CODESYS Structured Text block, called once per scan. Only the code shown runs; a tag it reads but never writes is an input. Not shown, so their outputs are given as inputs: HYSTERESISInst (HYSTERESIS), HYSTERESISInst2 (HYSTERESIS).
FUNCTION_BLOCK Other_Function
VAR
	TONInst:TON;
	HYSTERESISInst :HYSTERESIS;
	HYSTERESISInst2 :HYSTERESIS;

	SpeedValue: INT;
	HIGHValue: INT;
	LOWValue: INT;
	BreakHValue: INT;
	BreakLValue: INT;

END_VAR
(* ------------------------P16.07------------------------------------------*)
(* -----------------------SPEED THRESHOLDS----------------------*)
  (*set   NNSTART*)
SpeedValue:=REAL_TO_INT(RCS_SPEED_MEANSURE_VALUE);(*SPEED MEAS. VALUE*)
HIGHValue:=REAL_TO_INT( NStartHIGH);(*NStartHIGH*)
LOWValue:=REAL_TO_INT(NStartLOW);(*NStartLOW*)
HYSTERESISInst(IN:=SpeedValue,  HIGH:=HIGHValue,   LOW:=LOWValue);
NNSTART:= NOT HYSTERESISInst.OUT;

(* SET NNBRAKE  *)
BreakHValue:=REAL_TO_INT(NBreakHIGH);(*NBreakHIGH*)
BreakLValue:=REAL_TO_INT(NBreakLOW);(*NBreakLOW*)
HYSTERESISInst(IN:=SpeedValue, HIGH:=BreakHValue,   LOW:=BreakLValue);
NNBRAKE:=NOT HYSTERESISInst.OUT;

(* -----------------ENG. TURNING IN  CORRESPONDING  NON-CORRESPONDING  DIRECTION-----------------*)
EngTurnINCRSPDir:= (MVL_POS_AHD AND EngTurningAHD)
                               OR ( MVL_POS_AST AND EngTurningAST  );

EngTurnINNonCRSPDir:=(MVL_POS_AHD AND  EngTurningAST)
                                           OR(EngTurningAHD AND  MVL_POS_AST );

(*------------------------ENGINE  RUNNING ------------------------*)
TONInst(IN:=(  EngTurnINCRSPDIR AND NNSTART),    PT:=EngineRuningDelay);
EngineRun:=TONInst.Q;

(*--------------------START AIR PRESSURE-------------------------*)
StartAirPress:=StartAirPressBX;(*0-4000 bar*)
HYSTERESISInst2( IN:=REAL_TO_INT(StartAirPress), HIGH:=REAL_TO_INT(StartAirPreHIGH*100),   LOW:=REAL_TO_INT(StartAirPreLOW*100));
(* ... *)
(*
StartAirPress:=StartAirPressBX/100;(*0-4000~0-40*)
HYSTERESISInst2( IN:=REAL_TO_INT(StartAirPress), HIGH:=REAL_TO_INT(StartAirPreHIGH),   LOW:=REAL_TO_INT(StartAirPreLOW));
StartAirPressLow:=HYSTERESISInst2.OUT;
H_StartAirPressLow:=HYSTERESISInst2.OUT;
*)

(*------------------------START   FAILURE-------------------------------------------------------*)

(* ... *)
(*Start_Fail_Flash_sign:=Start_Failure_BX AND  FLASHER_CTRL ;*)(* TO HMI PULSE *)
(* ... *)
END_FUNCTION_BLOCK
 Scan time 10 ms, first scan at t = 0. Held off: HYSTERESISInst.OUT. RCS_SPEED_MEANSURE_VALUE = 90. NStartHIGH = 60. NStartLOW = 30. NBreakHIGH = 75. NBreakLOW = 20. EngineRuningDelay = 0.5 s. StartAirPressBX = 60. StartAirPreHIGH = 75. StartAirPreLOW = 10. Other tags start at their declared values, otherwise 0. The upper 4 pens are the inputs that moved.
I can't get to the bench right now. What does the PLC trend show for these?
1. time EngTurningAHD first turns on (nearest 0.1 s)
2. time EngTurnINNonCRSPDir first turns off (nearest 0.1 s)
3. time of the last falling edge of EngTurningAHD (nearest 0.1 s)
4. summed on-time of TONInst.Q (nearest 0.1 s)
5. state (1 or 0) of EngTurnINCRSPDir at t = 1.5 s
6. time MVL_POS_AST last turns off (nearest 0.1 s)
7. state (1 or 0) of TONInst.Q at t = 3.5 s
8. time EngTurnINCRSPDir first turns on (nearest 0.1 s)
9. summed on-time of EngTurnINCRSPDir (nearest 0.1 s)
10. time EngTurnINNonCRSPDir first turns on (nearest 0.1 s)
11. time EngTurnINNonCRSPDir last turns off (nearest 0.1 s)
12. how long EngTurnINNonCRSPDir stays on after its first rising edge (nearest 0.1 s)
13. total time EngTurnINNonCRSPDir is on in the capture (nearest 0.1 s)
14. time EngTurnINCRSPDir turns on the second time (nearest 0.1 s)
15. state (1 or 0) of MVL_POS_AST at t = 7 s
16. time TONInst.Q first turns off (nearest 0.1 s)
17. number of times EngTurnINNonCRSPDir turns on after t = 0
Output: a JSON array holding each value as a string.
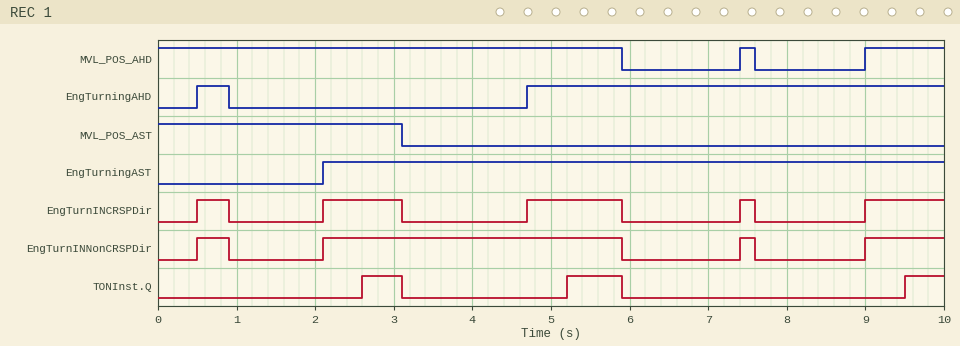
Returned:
["0.5 s", "0.9 s", "0.9 s", "1.7 s", "0", "3.1 s", "0", "0.5 s", "3.8 s", "0.5 s", "7.6 s", "0.4 s", "5.4 s", "2.1 s", "0", "3.1 s", "4"]
